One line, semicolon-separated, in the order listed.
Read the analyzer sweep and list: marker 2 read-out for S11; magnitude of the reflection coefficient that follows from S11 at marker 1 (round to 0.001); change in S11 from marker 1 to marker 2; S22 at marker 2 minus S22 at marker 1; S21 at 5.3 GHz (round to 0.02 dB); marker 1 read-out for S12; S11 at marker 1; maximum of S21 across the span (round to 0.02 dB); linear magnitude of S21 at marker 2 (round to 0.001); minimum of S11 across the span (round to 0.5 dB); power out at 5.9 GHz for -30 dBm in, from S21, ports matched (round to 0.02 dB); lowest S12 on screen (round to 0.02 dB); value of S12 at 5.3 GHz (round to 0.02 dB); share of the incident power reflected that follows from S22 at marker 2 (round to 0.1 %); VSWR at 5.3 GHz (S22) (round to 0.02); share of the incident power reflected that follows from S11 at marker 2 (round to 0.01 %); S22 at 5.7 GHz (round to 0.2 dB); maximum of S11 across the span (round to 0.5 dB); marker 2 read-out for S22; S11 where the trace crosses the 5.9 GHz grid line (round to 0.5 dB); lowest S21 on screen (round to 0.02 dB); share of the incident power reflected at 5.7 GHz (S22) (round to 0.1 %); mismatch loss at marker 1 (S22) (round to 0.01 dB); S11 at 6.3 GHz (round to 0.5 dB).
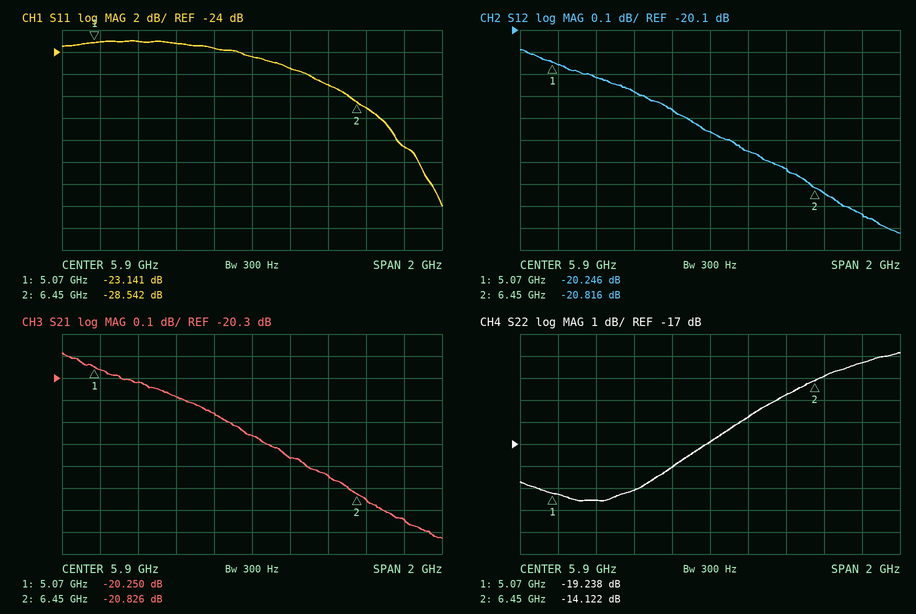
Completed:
-28.542 dB; 0.070; -5.401 dB; 5.116 dB; -20.32 dB; -20.246 dB; -23.141 dB; -20.18 dB; 0.091; -38.0 dB; -50.56 dBm; -21.02 dB; -20.32 dB; 3.9 %; 1.24; 0.14 %; -18.0 dB; -23.0 dB; -14.122 dB; -24.5 dB; -21.02 dB; 1.6 %; 0.05 dB; -27.0 dB
